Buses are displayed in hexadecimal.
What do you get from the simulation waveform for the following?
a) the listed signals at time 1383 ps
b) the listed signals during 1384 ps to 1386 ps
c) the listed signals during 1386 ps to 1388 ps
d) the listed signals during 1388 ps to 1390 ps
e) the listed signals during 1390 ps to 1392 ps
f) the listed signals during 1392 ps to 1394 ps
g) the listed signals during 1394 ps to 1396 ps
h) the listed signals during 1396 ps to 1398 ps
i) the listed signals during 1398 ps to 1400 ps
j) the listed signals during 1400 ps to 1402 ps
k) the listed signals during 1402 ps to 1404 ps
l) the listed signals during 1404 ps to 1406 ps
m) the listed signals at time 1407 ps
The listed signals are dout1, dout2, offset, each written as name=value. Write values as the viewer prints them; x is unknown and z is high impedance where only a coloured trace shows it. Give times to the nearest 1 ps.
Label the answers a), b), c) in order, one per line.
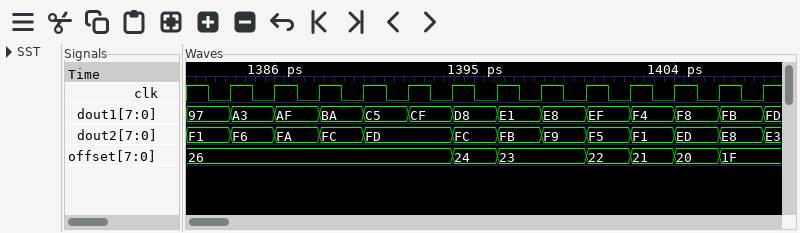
a) dout1=97, dout2=F1, offset=26
b) dout1=A3, dout2=F6, offset=26
c) dout1=AF, dout2=FA, offset=26
d) dout1=BA, dout2=FC, offset=26
e) dout1=C5, dout2=FD, offset=26
f) dout1=CF, dout2=FD, offset=26
g) dout1=D8, dout2=FC, offset=24
h) dout1=E1, dout2=FB, offset=23
i) dout1=E8, dout2=F9, offset=23
j) dout1=EF, dout2=F5, offset=22
k) dout1=F4, dout2=F1, offset=21
l) dout1=F8, dout2=ED, offset=20
m) dout1=FB, dout2=E8, offset=1F
